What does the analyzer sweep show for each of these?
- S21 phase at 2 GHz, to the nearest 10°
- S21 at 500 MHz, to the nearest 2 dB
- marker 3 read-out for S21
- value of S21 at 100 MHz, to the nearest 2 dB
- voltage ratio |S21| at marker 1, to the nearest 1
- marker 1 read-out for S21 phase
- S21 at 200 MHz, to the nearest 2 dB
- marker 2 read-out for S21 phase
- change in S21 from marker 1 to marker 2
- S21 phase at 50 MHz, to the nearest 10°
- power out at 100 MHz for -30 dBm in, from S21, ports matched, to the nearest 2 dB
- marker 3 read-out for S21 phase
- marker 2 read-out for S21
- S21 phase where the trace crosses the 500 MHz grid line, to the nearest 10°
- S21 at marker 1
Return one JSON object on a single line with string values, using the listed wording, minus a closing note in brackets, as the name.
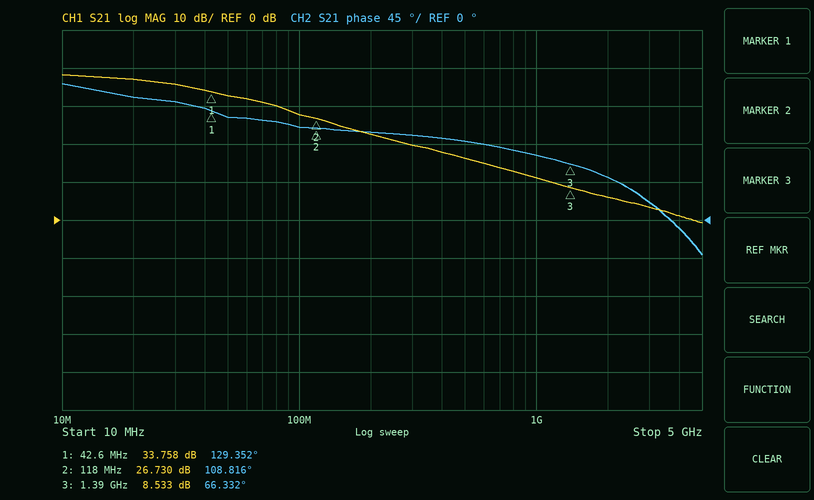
{"S21 phase at 2 GHz, to the nearest 10°": "50°", "S21 at 500 MHz, to the nearest 2 dB": "16 dB", "marker 3 read-out for S21": "8.533 dB", "value of S21 at 100 MHz, to the nearest 2 dB": "28 dB", "voltage ratio |S21| at marker 1, to the nearest 1": "49", "marker 1 read-out for S21 phase": "129.352°", "S21 at 200 MHz, to the nearest 2 dB": "22 dB", "marker 2 read-out for S21 phase": "108.816°", "change in S21 from marker 1 to marker 2": "-7.028 dB", "S21 phase at 50 MHz, to the nearest 10°": "120°", "power out at 100 MHz for -30 dBm in, from S21, ports matched, to the nearest 2 dB": "-2 dBm", "marker 3 read-out for S21 phase": "66.332°", "marker 2 read-out for S21": "26.730 dB", "S21 phase where the trace crosses the 500 MHz grid line, to the nearest 10°": "90°", "S21 at marker 1": "33.758 dB"}
